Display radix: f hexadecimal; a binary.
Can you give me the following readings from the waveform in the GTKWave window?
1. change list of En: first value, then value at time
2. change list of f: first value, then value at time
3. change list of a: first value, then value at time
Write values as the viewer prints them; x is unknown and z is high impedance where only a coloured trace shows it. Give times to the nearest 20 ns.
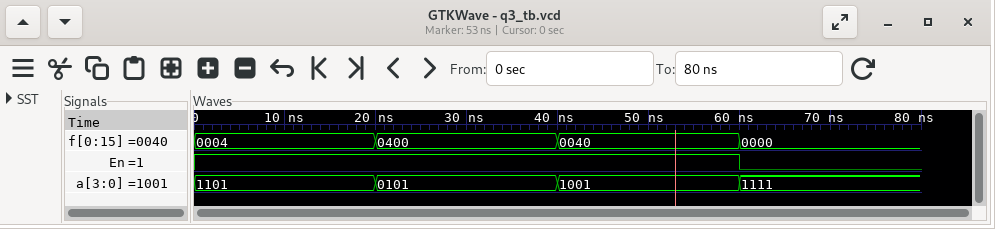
1, 0 at 60 ns
0004, 0400 at 20 ns, 0040 at 40 ns, 0000 at 60 ns
1101, 0101 at 20 ns, 1001 at 40 ns, 1111 at 60 ns
